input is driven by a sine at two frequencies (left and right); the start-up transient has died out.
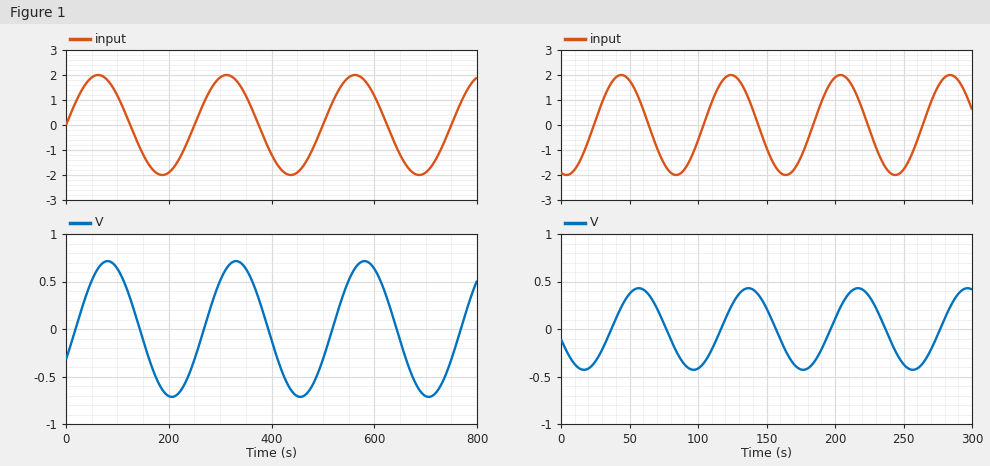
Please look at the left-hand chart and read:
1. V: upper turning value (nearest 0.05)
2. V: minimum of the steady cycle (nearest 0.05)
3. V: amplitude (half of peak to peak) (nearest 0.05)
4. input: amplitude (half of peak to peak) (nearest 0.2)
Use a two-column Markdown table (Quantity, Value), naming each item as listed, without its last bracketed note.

| Quantity | Value |
|---|---|
| V: upper turning value | 0.70 |
| V: minimum of the steady cycle | -0.70 |
| V: amplitude (half of peak to peak) | 0.70 |
| input: amplitude (half of peak to peak) | 2.0 |
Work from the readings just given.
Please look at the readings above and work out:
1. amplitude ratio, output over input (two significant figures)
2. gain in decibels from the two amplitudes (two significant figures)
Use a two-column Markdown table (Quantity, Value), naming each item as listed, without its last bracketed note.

| Quantity | Value |
|---|---|
| amplitude ratio, output over input | 0.35 |
| gain in decibels from the two amplitudes | -9.1 dB |
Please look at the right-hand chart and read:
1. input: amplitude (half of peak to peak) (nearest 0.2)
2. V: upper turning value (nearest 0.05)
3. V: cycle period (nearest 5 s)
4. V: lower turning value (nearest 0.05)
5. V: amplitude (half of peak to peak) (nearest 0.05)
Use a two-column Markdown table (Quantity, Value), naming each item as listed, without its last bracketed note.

| Quantity | Value |
|---|---|
| input: amplitude (half of peak to peak) | 2.0 |
| V: upper turning value | 0.45 |
| V: cycle period | 80 s |
| V: lower turning value | -0.45 |
| V: amplitude (half of peak to peak) | 0.45 |
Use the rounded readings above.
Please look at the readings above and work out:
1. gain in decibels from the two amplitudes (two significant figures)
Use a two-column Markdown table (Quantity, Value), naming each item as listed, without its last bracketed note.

| Quantity | Value |
|---|---|
| gain in decibels from the two amplitudes | -13 dB |
